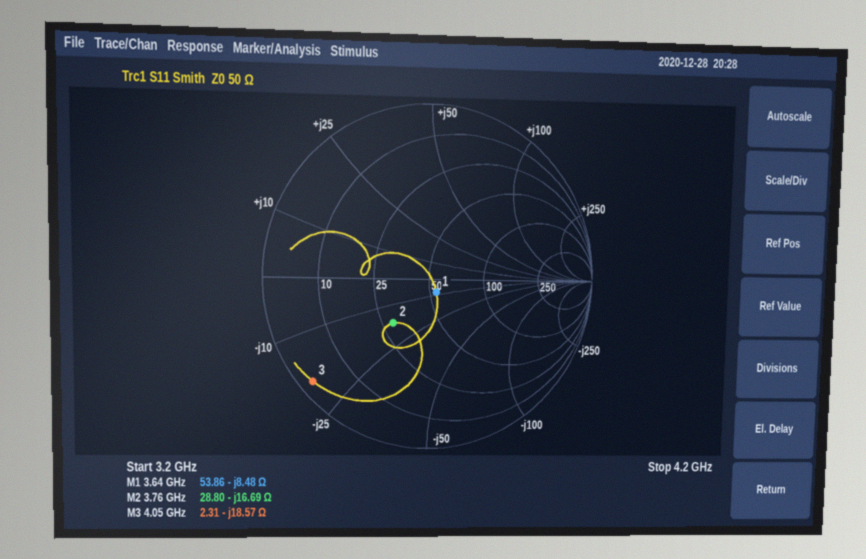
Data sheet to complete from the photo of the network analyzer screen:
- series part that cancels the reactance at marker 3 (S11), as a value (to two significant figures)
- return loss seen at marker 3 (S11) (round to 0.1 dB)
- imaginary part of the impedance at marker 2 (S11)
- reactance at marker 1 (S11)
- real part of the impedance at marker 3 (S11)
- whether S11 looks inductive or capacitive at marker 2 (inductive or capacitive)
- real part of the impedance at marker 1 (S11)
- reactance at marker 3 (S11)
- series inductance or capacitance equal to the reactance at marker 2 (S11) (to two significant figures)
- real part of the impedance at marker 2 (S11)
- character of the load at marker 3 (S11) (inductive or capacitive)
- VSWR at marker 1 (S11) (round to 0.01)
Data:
730 pH
0.7 dB
-16.69 Ω
-8.48 Ω
2.31 Ω
capacitive
53.86 Ω
-18.57 Ω
2.5 pF
28.80 Ω
capacitive
1.20
